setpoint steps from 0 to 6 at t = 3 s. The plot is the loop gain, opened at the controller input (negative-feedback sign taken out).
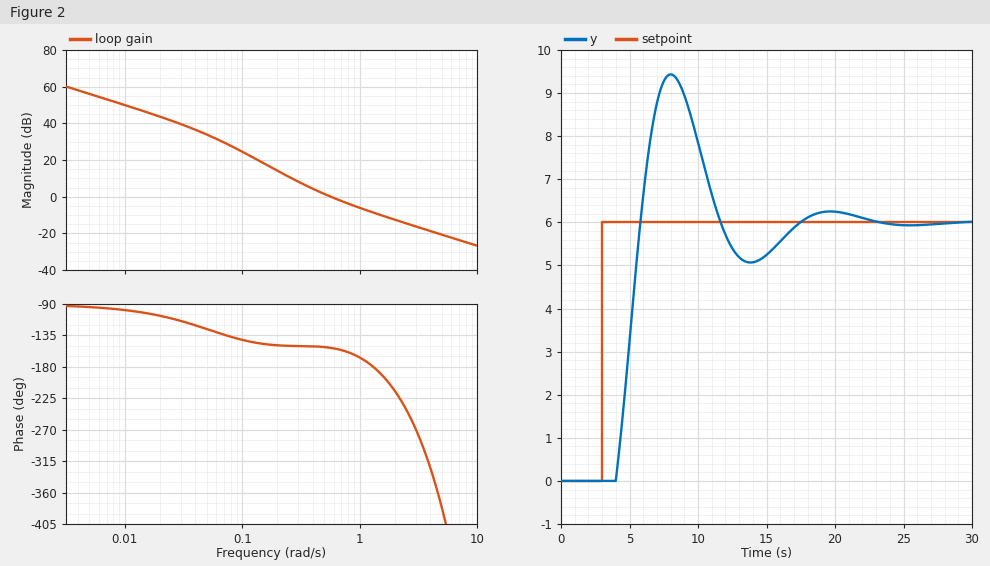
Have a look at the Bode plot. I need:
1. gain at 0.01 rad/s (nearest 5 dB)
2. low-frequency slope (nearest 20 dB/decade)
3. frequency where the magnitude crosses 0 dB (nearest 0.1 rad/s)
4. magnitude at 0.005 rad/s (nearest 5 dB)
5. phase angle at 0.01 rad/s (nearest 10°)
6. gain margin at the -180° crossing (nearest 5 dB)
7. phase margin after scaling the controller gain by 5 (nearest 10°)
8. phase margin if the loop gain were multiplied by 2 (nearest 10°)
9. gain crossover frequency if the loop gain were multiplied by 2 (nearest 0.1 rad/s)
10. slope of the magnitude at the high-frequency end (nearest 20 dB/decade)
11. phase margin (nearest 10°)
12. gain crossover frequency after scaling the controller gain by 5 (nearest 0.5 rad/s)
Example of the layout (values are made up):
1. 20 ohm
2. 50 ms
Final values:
1. 50 dB
2. -20 dB/decade
3. 0.6 rad/s
4. 55 dB
5. -100°
6. 10 dB
7. -50°
8. 10°
9. 1.0 rad/s
10. -20 dB/decade
11. 30°
12. 2.5 rad/s
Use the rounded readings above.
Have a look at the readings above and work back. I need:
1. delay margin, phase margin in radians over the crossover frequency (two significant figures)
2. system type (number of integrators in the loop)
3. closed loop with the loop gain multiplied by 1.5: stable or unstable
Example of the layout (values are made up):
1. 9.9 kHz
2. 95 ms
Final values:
1. 0.87 s
2. 1
3. stable
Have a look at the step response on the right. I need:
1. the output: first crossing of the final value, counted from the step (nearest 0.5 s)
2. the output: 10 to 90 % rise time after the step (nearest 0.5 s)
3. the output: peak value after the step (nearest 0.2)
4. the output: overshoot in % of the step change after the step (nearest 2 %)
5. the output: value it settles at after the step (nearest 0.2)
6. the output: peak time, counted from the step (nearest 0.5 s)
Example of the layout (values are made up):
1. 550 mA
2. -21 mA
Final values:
1. 3.0 s
2. 1.5 s
3. 9.4
4. 58 %
5. 6.0
6. 5.0 s
